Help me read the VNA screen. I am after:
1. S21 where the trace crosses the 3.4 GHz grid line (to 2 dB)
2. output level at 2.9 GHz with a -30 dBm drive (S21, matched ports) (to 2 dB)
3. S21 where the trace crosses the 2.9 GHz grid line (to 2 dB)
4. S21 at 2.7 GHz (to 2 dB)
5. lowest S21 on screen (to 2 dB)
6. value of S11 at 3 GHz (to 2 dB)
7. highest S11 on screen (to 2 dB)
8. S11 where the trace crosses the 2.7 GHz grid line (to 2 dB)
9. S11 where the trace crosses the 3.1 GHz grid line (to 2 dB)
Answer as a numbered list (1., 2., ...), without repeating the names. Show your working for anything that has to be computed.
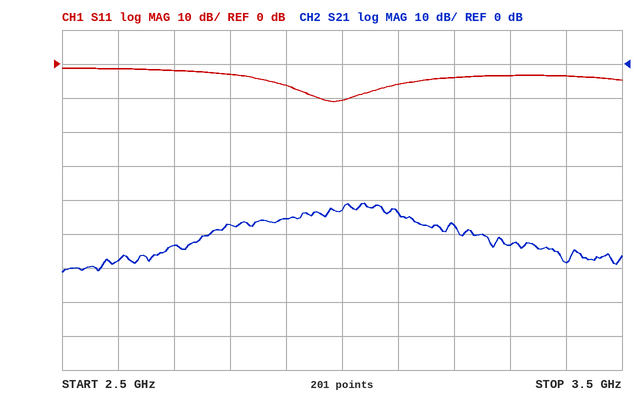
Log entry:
1. -58 dB
2. -30 dBm + (-46 dB) = -76 dBm
3. -46 dB
4. -54 dB
5. -62 dB
6. -10 dB
7. -2 dB
8. -2 dB
9. -6 dB
